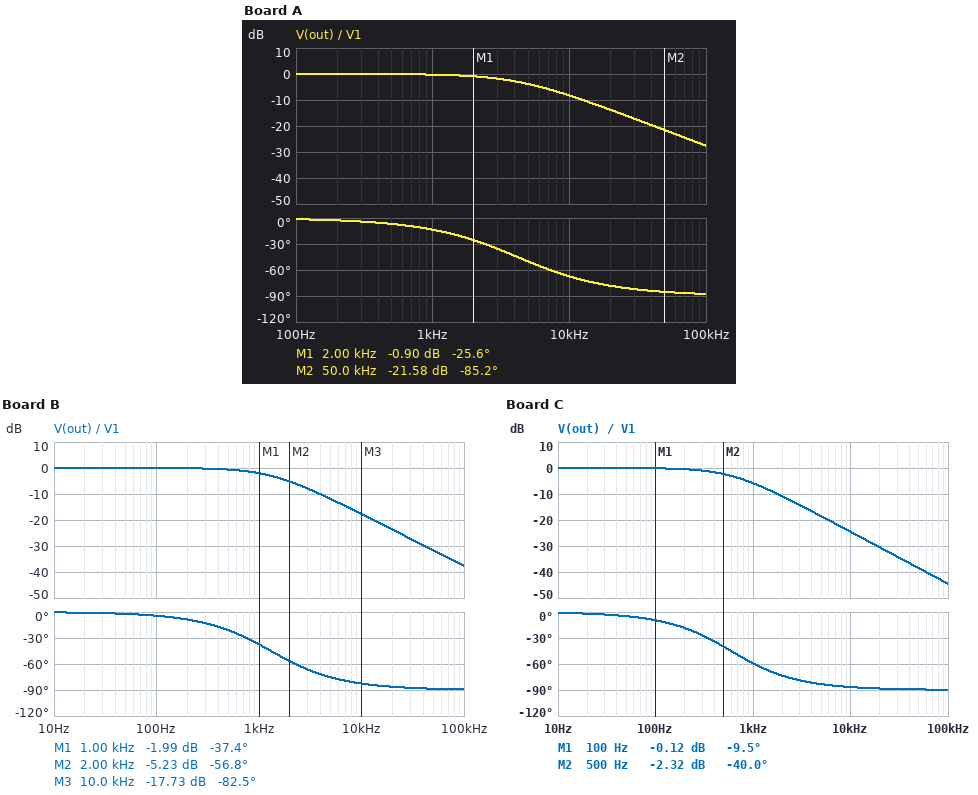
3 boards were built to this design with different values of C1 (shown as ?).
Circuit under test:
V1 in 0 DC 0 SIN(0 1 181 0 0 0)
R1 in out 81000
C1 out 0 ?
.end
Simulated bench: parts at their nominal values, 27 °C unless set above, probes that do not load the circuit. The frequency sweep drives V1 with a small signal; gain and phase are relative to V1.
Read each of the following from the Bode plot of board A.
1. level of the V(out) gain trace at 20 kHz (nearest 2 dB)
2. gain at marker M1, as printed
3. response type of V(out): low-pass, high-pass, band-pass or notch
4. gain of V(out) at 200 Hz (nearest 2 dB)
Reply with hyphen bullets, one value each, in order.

- -14 dB
- -0.90 dB
- low-pass
- 0 dB
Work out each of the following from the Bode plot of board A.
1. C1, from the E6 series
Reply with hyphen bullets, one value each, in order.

- 470 pF
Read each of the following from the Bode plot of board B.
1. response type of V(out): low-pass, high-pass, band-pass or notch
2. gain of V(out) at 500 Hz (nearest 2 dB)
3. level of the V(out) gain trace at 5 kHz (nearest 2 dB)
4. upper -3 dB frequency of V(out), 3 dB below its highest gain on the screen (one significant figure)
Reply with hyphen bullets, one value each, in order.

- low-pass
- 0 dB
- -12 dB
- 1 kHz
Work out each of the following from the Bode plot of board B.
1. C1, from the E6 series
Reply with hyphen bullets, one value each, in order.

- 1.5 nF
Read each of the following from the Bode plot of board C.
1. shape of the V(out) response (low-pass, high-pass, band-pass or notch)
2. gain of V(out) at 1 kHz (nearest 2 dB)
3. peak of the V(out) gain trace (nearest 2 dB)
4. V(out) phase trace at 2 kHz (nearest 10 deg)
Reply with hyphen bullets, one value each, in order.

- low-pass
- -6 dB
- 0 dB
- -70 deg
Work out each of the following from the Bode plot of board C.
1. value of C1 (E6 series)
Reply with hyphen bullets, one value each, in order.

- 3.3 nF
